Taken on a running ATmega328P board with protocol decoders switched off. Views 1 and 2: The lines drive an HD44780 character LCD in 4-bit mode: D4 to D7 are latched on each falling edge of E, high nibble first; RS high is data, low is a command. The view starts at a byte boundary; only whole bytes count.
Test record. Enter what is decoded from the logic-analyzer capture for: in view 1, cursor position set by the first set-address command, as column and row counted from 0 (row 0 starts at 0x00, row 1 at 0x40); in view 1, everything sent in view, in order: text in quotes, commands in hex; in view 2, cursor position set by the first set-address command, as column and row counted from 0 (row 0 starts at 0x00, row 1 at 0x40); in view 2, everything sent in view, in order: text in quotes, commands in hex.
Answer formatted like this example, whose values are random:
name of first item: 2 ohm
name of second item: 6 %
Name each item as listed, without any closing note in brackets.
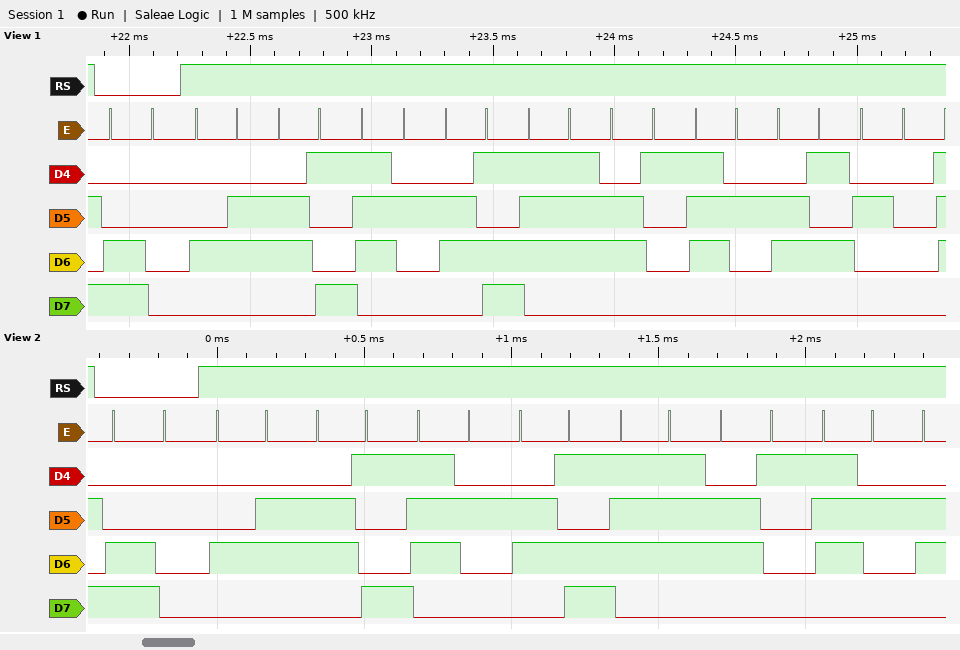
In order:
in view 1, cursor position set by the first set-address command, as column and row counted from 0: column 0, row 1
in view 1, everything sent in view, in order: text in quotes, commands in hex: 0xC0 "Firmware "
in view 2, cursor position set by the first set-address command, as column and row counted from 0: column 0, row 1
in view 2, everything sent in view, in order: text in quotes, commands in hex: 0xC0 "Firmwar"
